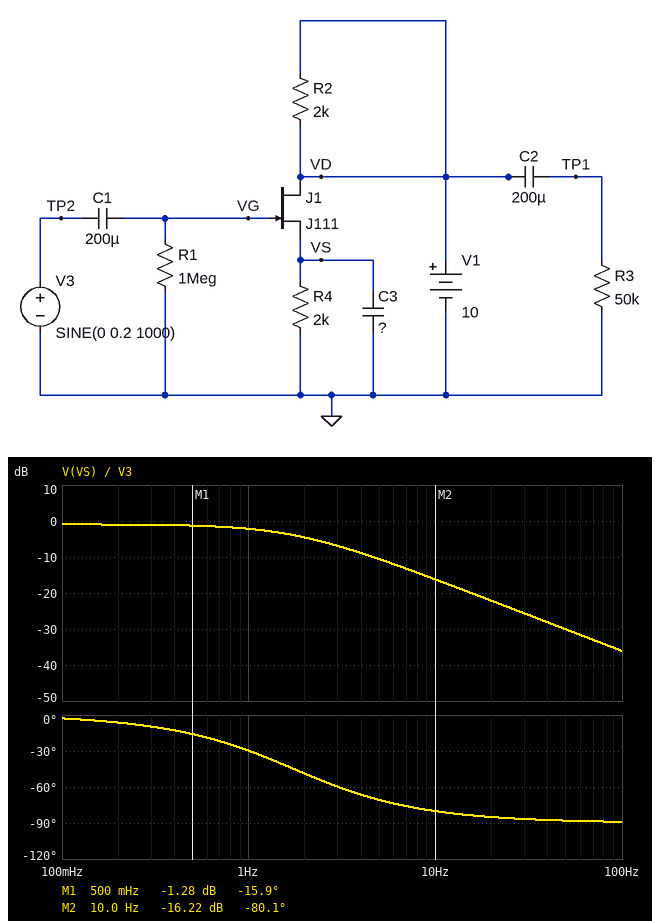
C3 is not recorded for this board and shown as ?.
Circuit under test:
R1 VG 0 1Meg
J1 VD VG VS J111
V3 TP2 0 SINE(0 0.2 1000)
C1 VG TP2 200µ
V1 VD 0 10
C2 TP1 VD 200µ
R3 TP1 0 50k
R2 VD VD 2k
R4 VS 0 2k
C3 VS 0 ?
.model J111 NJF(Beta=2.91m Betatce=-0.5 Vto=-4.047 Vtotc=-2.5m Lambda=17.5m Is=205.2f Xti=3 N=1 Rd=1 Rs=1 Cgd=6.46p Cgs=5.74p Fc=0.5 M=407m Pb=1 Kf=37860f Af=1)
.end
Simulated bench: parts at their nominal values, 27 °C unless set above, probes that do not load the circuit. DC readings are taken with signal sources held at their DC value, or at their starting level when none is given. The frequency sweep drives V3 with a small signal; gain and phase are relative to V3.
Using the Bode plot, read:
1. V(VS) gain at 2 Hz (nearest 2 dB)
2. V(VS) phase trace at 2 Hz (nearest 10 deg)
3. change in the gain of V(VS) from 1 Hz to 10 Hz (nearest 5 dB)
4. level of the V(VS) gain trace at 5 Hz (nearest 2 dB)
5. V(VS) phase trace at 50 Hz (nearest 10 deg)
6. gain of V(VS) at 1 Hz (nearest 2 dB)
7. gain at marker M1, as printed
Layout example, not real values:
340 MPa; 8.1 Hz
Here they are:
-4 dB; -50 deg; -15 dB; -10 dB; -90 deg; -2 dB; -1.28 dB
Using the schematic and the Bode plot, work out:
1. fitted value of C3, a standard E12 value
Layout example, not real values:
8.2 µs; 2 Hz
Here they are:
470 µF
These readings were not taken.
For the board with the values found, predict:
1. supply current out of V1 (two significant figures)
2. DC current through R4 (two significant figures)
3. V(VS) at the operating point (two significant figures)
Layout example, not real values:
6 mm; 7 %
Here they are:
1.7 mA; 1.7 mA; 3.3 V
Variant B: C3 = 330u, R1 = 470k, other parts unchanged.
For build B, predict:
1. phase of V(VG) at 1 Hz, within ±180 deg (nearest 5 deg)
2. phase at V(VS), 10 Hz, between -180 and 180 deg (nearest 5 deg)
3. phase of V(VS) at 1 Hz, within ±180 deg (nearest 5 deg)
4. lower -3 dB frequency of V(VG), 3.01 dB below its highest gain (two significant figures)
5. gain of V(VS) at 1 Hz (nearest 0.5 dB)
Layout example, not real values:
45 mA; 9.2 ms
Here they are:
0 deg; -75 deg; -20 deg; 1.7 mHz; -1.5 dB
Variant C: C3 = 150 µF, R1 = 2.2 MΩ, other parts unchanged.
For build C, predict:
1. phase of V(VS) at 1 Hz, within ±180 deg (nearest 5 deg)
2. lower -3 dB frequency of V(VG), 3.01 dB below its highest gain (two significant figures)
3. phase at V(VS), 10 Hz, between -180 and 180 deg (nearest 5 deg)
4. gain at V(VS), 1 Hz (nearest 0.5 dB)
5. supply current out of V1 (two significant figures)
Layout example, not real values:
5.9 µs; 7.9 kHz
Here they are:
-10 deg; 360 µHz; -60 deg; -1.0 dB; 1.7 mA
